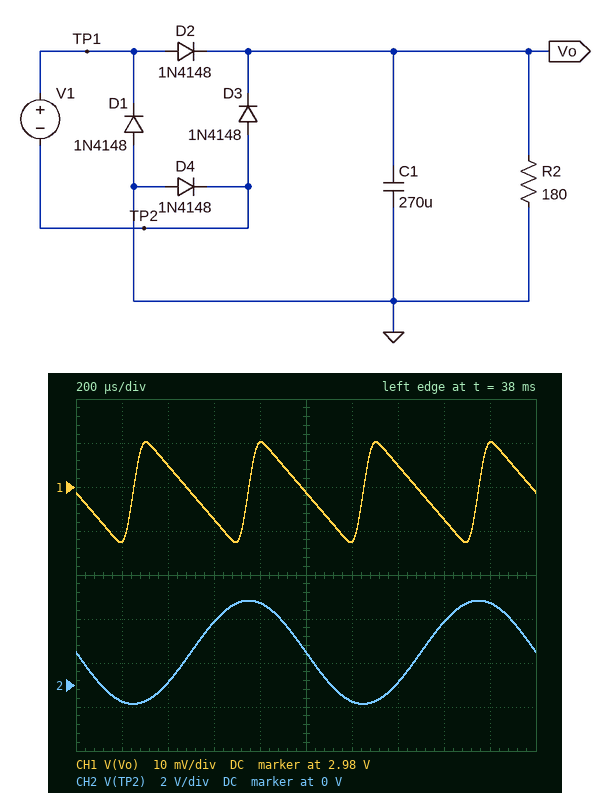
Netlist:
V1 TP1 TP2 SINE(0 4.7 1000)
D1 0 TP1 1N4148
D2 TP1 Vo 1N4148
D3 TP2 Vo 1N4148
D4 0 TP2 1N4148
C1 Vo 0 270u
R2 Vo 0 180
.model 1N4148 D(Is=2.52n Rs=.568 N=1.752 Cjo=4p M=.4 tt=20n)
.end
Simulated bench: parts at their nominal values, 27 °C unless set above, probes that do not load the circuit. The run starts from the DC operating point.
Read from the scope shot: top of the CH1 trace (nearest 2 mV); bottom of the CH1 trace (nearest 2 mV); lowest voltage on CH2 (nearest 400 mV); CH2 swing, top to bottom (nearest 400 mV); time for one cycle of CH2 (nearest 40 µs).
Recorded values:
2.990 V
2.968 V
-800 mV
4.8 V
1.00 ms
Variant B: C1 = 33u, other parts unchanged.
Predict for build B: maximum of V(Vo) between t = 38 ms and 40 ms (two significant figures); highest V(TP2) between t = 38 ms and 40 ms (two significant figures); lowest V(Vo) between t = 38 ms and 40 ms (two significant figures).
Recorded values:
3.1 V
3.9 V
2.9 V
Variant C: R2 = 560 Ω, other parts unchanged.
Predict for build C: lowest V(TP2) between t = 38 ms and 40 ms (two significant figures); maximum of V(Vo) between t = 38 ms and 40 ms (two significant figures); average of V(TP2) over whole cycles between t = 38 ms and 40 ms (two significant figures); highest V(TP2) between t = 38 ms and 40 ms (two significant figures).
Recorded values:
-780 mV
3.1 V
1.6 V
3.9 V
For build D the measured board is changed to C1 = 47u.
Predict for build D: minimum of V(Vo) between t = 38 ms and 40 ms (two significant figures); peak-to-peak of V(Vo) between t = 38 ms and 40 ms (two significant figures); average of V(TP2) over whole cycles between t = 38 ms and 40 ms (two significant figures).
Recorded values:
2.9 V
130 mV
1.5 V
